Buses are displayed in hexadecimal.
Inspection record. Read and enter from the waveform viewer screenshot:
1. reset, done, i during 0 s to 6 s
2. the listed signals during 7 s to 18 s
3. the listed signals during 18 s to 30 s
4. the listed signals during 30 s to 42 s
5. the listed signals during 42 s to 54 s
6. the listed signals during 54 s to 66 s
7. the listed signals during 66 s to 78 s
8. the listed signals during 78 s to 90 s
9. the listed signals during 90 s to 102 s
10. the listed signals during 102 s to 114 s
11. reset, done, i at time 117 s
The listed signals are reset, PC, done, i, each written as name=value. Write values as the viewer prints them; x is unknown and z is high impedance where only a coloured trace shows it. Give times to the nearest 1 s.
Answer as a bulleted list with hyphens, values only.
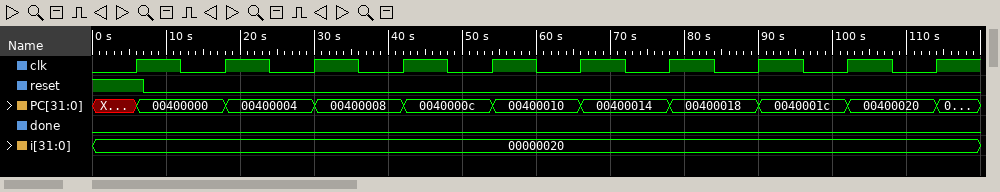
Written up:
- reset=1, done=0, i=00000020
- reset=0, PC=00400000, done=0, i=00000020
- reset=0, PC=00400004, done=0, i=00000020
- reset=0, PC=00400008, done=0, i=00000020
- reset=0, PC=0040000c, done=0, i=00000020
- reset=0, PC=00400010, done=0, i=00000020
- reset=0, PC=00400014, done=0, i=00000020
- reset=0, PC=00400018, done=0, i=00000020
- reset=0, PC=0040001c, done=0, i=00000020
- reset=0, PC=00400020, done=0, i=00000020
- reset=0, done=0, i=00000020
